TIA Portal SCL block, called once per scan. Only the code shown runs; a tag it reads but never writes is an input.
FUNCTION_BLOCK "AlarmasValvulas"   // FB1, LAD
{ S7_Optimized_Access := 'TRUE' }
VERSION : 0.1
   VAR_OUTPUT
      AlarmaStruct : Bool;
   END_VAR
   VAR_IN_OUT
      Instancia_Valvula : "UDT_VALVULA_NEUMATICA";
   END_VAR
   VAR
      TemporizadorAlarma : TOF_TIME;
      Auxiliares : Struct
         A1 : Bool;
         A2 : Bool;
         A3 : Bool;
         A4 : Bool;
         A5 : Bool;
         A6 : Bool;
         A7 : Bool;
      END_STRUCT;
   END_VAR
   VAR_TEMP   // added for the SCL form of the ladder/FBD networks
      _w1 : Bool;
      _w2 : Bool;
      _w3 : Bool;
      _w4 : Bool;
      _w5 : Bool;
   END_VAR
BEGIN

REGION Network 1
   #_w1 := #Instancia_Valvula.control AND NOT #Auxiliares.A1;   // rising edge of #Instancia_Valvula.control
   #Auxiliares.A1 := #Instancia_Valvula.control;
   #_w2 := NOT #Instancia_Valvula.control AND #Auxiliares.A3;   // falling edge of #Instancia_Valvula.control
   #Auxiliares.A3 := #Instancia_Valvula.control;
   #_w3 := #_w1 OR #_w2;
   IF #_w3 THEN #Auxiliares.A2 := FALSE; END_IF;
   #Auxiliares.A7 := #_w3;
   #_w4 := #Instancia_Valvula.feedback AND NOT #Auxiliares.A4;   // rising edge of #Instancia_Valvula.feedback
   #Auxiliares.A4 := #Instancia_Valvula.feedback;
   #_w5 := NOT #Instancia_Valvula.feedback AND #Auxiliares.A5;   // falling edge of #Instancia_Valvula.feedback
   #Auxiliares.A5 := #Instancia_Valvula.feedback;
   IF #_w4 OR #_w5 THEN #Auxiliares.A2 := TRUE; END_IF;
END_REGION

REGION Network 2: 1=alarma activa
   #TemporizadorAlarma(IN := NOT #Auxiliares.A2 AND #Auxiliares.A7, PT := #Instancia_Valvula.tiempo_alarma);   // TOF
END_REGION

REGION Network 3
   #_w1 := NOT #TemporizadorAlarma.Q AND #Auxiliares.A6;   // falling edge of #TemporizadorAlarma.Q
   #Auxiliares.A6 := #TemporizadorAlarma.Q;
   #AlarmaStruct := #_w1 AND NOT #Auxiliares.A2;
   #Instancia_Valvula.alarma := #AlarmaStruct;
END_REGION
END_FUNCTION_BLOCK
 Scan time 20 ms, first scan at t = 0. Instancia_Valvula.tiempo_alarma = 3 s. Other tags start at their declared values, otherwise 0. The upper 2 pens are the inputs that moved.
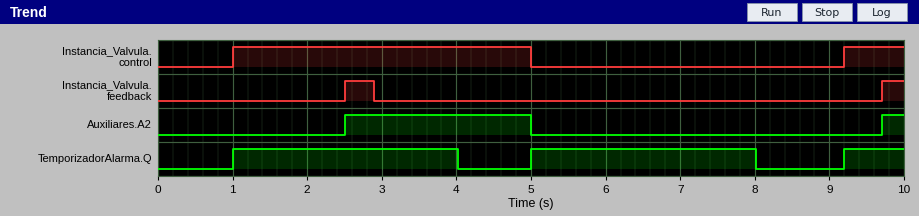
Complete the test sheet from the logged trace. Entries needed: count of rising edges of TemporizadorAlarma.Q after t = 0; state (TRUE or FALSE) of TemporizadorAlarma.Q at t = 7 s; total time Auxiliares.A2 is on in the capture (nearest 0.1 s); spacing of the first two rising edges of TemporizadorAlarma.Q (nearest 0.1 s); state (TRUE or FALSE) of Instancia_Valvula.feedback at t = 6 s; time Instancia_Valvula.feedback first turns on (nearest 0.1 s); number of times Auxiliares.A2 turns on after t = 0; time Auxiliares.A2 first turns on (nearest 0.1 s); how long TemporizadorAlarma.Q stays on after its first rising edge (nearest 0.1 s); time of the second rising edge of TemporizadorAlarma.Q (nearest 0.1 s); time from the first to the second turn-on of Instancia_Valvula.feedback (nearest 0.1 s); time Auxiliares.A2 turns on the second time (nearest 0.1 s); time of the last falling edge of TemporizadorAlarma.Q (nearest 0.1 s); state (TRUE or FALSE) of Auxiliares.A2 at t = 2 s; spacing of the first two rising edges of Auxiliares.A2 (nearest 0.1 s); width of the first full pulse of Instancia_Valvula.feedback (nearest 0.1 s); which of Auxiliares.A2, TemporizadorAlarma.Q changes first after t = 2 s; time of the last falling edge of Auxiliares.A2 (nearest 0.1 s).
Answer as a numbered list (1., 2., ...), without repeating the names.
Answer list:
1. 3
2. TRUE
3. 2.8 s
4. 4.0 s
5. FALSE
6. 2.5 s
7. 2
8. 2.5 s
9. 3.0 s
10. 5.0 s
11. 7.2 s
12. 9.7 s
13. 8.0 s
14. FALSE
15. 7.2 s
16. 0.4 s
17. Auxiliares.A2
18. 5.0 s
